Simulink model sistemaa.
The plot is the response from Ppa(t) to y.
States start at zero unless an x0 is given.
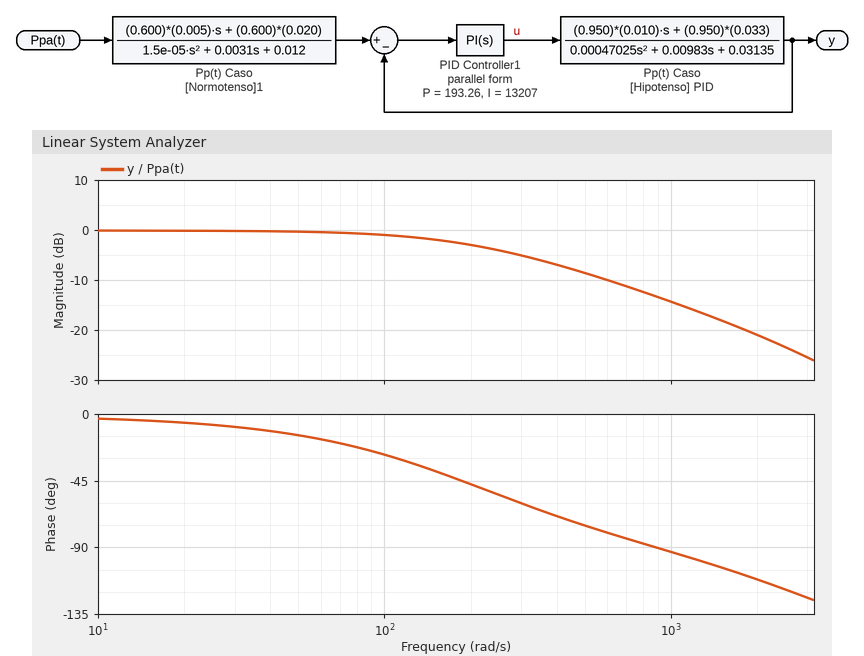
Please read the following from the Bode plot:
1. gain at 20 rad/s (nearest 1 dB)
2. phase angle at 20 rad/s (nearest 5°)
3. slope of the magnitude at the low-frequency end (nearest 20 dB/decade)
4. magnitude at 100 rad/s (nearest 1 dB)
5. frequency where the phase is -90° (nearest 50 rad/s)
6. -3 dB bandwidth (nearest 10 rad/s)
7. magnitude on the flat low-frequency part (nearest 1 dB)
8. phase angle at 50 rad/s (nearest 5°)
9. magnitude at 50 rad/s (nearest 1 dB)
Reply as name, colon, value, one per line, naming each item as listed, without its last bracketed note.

gain at 20 rad/s: 0 dB
phase angle at 20 rad/s: -5°
slope of the magnitude at the low-frequency end: 0 dB/decade
magnitude at 100 rad/s: -1 dB
frequency where the phase is -90°: 900 rad/s
-3 dB bandwidth: 210 rad/s
magnitude on the flat low-frequency part: 0 dB
phase angle at 50 rad/s: -15°
magnitude at 50 rad/s: 0 dB
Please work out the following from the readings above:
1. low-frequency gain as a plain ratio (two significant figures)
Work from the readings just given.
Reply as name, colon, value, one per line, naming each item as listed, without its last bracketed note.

low-frequency gain as a plain ratio: 1.0
